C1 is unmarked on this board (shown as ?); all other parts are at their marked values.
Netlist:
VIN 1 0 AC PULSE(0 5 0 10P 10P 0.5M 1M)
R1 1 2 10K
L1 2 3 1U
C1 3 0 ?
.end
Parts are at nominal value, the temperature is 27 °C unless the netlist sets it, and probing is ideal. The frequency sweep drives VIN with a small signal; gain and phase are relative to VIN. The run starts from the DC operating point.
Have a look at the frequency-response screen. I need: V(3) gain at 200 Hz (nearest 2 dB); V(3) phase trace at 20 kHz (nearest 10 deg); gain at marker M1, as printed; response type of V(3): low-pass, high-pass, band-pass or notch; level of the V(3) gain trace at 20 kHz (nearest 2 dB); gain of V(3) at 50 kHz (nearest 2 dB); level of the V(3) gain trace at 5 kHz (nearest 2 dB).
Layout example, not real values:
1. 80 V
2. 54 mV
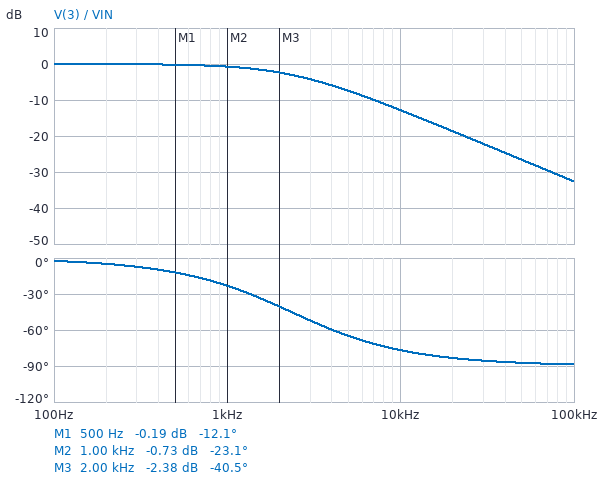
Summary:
1. 0 dB
2. -80 deg
3. -0.19 dB
4. low-pass
5. -18 dB
6. -26 dB
7. -8 dB
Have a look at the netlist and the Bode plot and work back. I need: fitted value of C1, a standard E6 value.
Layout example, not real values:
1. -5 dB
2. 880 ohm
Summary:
1. 6.8 nF
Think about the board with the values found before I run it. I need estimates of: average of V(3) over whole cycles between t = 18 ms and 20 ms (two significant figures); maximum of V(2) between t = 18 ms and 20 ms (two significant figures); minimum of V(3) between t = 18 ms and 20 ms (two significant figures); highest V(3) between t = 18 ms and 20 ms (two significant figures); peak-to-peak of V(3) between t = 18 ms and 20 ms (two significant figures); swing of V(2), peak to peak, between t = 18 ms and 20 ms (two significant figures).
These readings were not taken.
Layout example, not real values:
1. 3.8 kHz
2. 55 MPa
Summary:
1. 2.5 V
2. 5.0 V
3. 3.2 mV
4. 5.0 V
5. 5.0 V
6. 5.0 V
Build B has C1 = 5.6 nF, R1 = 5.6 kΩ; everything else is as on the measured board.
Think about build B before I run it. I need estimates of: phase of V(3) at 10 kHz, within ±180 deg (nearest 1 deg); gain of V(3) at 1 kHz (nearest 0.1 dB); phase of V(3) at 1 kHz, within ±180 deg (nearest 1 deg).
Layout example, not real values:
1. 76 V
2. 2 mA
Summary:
1. -63 deg
2. -0.2 dB
3. -11 deg
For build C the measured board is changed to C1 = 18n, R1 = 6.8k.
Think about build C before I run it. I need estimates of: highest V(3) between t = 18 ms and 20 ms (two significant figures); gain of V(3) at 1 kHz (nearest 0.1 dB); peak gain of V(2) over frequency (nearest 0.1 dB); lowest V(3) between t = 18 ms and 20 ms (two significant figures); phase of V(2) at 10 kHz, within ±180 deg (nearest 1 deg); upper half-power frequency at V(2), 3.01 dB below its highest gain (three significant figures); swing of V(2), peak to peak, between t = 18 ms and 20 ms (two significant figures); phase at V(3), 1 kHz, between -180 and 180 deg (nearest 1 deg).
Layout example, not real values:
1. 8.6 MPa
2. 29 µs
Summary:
1. 4.9 V
2. -2.0 dB
3. 0 dB
4. 83 mV
5. -83 deg
6. 1.30 kHz
7. 4.8 V
8. -38 deg
